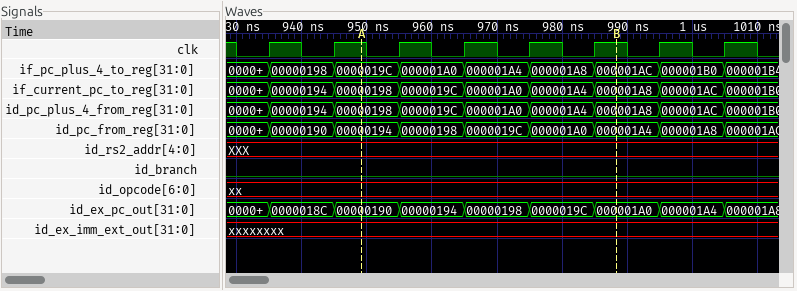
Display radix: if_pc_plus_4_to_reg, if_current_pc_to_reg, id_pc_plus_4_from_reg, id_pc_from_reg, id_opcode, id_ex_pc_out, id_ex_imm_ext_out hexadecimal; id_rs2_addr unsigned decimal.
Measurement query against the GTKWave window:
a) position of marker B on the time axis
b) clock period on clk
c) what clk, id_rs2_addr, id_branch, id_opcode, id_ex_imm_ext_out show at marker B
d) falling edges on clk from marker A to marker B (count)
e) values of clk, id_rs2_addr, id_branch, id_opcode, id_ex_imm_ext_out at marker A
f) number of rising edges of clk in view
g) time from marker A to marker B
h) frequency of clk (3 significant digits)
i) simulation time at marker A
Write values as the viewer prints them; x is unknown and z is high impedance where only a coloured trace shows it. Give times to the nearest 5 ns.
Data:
990 ns
10 ns
clk=1, id_rs2_addr=XXX, id_branch=0, id_opcode=xx, id_ex_imm_ext_out=xxxxxxxx
4
clk=1, id_rs2_addr=XXX, id_branch=0, id_opcode=xx, id_ex_imm_ext_out=xxxxxxxx
8
40 ns
100 MHz
950 ns
